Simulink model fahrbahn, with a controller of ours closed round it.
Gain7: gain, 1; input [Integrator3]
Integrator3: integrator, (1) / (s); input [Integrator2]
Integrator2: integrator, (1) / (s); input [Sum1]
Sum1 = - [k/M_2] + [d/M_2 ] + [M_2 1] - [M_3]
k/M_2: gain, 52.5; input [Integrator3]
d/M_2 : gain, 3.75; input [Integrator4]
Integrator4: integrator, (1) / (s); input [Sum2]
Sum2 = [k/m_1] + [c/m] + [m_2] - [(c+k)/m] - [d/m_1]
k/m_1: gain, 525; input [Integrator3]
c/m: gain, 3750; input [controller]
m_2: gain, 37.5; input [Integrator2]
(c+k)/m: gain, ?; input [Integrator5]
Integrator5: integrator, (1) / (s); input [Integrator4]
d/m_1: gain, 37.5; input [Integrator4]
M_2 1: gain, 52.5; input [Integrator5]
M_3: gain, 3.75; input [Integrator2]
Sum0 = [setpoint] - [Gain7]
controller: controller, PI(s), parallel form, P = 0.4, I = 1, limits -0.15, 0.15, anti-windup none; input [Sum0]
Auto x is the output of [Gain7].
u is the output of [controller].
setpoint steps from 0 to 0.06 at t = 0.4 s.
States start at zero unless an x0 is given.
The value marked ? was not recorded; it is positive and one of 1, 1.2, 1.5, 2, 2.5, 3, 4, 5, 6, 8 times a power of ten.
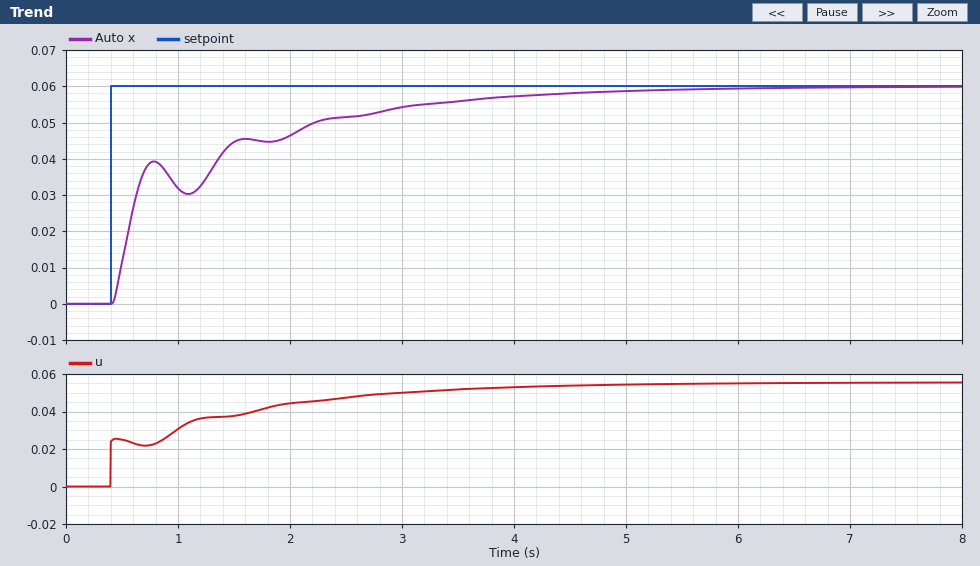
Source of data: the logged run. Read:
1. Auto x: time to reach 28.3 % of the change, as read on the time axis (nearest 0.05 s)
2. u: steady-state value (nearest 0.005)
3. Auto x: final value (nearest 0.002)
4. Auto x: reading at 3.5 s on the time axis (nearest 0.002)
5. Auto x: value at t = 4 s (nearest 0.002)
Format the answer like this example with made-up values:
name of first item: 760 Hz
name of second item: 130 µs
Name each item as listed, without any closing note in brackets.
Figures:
Auto x: time to reach 28.3 % of the change, as read on the time axis: 0.55 s
u: steady-state value: 0.055
Auto x: final value: 0.060
Auto x: reading at 3.5 s on the time axis: 0.056
Auto x: value at t = 4 s: 0.058
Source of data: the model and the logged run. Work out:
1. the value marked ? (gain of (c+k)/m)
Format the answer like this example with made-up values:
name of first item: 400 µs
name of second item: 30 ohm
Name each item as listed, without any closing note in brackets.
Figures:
the value marked ? (gain of (c+k)/m): 4000
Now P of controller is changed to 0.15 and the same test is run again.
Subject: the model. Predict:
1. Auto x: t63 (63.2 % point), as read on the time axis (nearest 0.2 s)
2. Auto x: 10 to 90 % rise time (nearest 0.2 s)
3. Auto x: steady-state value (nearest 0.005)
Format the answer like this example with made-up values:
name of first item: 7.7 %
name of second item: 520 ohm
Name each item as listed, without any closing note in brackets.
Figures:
Auto x: t63 (63.2 % point), as read on the time axis: 1.4 s
Auto x: 10 to 90 % rise time: 2.0 s
Auto x: steady-state value: 0.060
